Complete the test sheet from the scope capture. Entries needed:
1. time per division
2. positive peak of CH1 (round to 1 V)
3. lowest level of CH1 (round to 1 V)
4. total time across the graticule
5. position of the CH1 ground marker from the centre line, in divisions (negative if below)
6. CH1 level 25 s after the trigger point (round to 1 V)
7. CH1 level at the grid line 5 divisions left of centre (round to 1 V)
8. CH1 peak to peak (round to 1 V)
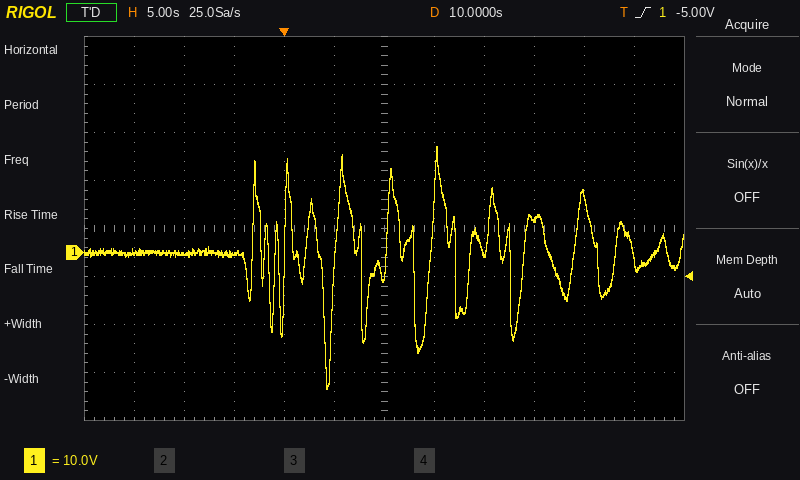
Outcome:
5 s
22 V
-28 V
60 s
-0.5 div
7 V
0 V
50 V
